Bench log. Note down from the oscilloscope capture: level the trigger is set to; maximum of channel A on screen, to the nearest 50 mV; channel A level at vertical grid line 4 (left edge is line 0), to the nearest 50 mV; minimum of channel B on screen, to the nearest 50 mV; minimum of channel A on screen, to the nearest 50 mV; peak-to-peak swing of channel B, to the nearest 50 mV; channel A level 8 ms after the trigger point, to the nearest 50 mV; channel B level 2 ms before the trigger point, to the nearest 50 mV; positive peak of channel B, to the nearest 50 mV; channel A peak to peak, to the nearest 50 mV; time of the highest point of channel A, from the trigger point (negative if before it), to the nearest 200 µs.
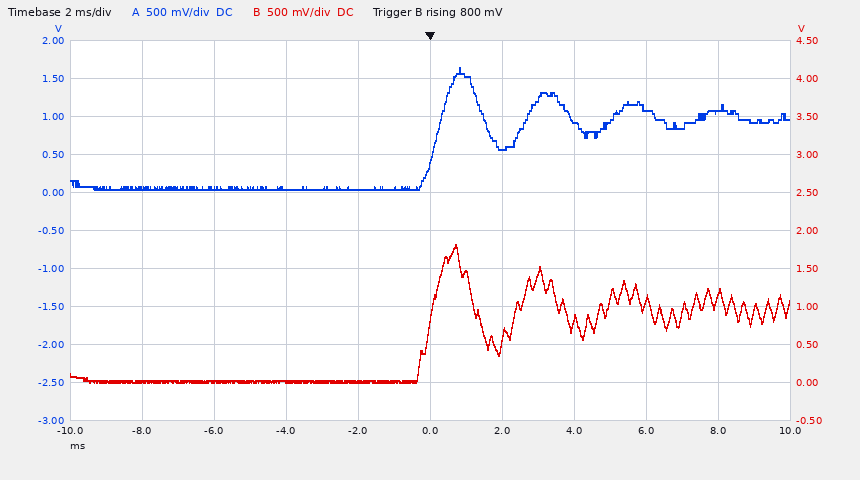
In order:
800 mV
1.65 V
50 mV
0 mV
50 mV
1.80 V
1.05 V
0 mV
1.80 V
1.60 V
+800 µs
